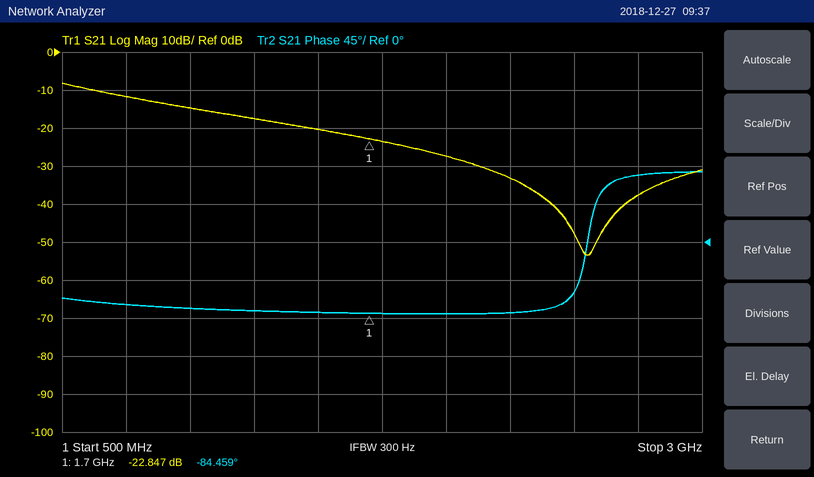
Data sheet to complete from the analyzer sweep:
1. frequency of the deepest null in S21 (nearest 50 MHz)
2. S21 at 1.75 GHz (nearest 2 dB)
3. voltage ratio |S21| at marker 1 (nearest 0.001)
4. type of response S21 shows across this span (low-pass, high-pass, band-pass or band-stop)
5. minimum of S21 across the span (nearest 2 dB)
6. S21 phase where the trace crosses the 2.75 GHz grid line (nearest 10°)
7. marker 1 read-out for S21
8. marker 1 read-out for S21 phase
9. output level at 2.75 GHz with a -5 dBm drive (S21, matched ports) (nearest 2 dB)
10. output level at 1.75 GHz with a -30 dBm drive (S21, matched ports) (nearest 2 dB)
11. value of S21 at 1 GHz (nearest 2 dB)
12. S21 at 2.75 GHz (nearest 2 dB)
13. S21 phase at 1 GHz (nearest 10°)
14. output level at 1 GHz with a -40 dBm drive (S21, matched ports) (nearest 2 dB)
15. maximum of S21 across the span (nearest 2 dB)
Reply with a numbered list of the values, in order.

1. 2.55 GHz
2. -24 dB
3. 0.072
4. low-pass
5. -54 dB
6. 80°
7. -22.847 dB
8. -84.459°
9. -42 dBm
10. -54 dBm
11. -14 dB
12. -38 dB
13. -80°
14. -54 dBm
15. -8 dB
